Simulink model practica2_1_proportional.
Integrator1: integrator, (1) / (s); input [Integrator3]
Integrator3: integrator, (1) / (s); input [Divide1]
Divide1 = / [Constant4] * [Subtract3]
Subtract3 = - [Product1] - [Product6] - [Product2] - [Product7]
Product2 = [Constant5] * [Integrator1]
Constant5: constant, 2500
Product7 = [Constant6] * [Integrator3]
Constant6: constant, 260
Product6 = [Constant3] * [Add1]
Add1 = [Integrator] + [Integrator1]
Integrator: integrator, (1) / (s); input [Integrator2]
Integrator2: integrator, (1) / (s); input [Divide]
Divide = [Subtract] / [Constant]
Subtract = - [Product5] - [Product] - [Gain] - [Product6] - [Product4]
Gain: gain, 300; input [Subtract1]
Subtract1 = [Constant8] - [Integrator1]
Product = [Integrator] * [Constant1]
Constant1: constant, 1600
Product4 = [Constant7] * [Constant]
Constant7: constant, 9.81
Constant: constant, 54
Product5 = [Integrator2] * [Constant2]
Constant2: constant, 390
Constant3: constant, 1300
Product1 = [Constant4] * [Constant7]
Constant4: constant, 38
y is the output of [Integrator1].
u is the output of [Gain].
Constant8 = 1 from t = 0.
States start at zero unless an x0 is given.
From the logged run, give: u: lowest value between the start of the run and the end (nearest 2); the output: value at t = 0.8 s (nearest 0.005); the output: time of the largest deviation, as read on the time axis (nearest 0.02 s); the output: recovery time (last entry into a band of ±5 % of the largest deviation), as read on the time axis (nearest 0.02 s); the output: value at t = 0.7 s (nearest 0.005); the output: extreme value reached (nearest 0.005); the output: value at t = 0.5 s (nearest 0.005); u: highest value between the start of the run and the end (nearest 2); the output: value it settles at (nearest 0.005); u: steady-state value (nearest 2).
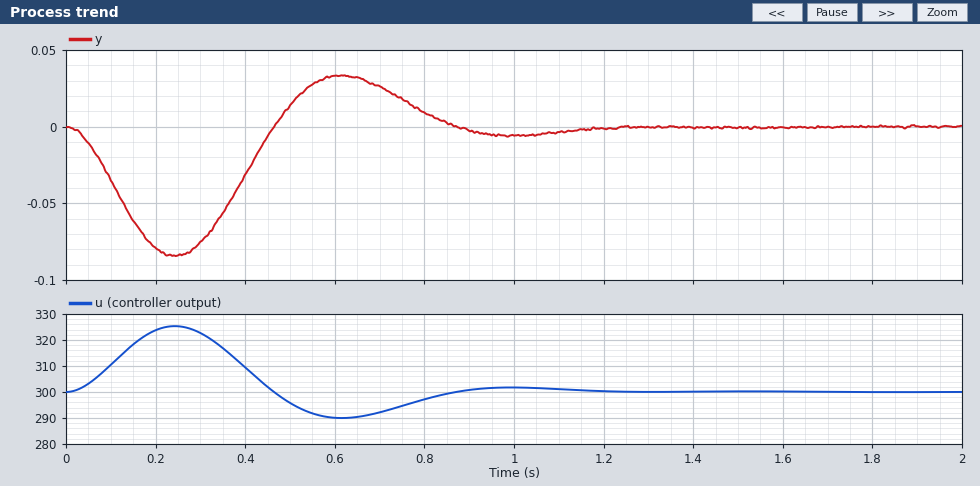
290
0.010
0.24 s
1.08 s
0.025
-0.085
0.015
326
0.000
300
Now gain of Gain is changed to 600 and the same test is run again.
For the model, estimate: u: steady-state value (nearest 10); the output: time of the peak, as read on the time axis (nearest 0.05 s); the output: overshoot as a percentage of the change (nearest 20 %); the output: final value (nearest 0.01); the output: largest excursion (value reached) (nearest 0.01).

580
0.60 s
120 %
0.04
0.09
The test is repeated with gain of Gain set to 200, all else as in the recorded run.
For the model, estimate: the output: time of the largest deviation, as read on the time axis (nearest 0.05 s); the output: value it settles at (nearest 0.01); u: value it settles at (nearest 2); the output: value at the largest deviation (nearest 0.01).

0.25 s
-0.01
202
-0.09
